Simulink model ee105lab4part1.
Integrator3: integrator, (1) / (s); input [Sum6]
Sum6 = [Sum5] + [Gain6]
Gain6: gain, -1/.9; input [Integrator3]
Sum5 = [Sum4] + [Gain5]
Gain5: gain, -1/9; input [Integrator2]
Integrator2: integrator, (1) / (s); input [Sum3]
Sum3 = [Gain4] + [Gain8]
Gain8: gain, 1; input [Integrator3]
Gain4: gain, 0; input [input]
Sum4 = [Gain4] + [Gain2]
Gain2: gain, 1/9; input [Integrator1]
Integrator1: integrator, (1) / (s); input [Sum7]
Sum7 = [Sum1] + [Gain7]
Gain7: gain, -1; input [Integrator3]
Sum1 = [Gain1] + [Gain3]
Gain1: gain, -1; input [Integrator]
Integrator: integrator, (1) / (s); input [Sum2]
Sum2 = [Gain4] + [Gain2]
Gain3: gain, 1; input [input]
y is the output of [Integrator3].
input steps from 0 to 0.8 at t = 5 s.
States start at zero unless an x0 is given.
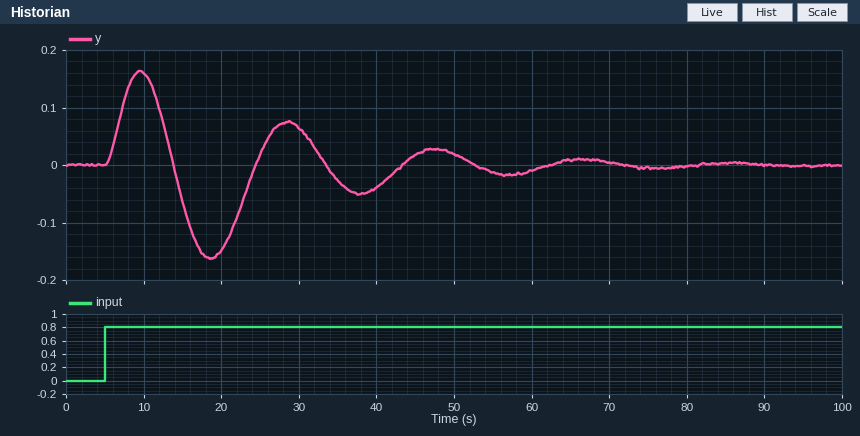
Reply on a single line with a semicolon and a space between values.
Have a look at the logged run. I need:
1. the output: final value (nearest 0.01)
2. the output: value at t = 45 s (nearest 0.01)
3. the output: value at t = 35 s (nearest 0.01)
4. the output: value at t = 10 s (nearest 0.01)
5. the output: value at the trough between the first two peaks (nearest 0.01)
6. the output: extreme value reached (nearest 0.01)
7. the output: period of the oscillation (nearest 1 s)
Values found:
0.00; 0.02; -0.03; 0.16; -0.16; 0.16; 19 s
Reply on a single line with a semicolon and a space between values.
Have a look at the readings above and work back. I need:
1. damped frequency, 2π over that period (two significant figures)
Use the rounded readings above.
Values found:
0.33 rad/s
